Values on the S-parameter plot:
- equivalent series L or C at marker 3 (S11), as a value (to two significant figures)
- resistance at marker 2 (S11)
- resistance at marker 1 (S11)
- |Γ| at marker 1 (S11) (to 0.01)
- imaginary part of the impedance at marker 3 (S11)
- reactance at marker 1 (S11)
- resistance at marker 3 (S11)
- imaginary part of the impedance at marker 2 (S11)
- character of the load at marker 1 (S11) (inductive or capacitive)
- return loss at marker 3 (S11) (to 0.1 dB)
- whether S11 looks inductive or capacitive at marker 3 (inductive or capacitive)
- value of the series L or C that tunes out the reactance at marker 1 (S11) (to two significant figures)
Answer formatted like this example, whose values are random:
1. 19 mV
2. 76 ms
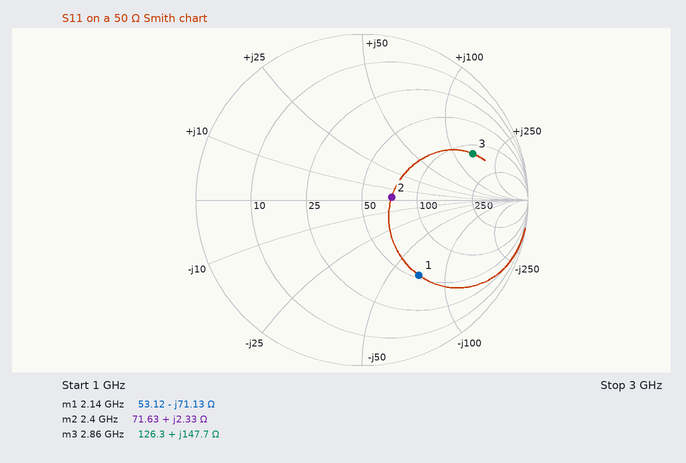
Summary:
1. 8.2 nH
2. 71.63 Ω
3. 53.12 Ω
4. 0.57
5. +147.7 Ω
6. -71.13 Ω
7. 126.3 Ω
8. +2.33 Ω
9. capacitive
10. 2.8 dB
11. inductive
12. 5.3 nH
